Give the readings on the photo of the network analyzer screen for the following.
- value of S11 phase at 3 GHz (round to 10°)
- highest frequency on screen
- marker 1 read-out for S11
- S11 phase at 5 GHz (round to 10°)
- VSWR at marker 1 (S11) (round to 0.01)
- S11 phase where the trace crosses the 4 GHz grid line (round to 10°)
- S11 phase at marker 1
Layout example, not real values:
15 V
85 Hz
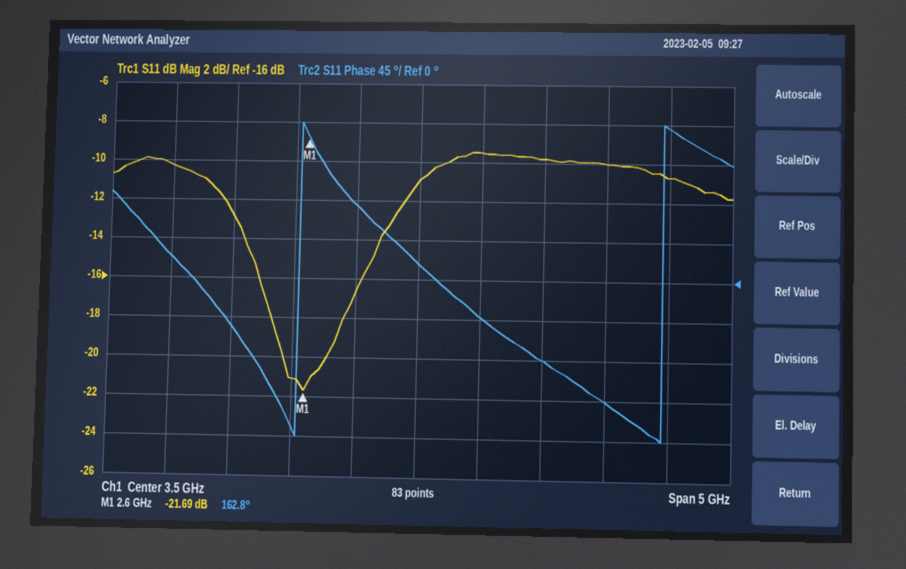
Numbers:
80°
6 GHz
-21.69 dB
-140°
1.18
-40°
162.8°
